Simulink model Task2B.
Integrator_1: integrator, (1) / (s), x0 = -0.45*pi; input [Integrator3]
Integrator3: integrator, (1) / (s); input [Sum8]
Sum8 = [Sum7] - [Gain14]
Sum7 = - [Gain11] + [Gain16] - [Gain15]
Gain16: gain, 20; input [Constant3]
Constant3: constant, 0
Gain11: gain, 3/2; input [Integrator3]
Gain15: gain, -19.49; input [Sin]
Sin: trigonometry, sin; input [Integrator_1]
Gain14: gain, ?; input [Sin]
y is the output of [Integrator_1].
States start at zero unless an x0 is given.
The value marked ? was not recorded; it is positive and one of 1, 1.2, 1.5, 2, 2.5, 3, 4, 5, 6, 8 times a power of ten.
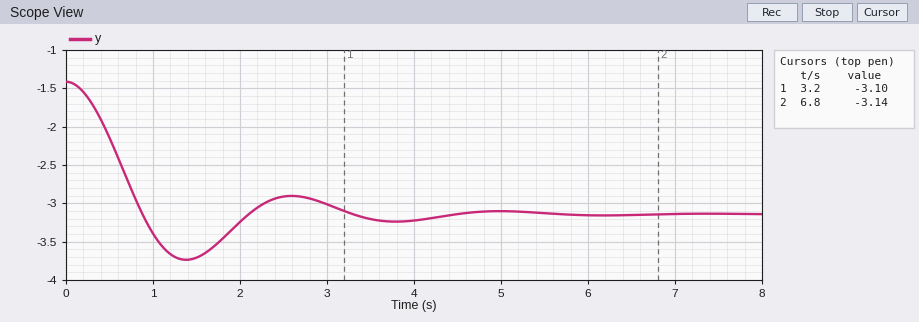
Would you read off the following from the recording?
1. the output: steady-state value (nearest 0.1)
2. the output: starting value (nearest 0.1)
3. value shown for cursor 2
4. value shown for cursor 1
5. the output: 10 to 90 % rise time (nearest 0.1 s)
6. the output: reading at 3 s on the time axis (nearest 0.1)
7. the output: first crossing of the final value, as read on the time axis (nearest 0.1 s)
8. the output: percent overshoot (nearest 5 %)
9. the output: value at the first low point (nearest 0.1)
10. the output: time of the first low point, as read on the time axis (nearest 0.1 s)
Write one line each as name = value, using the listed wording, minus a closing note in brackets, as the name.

the output: steady-state value = -3.1
the output: starting value = -1.4
value shown for cursor 2 = -3.14
value shown for cursor 1 = -3.10
the output: 10 to 90 % rise time = 0.6 s
the output: reading at 3 s on the time axis = -3.0
the output: first crossing of the final value, as read on the time axis = 0.9 s
the output: percent overshoot = 35 %
the output: value at the first low point = -3.7
the output: time of the first low point, as read on the time axis = 1.4 s
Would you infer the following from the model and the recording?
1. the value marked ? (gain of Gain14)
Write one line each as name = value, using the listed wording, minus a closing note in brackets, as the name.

the value marked ? = 12
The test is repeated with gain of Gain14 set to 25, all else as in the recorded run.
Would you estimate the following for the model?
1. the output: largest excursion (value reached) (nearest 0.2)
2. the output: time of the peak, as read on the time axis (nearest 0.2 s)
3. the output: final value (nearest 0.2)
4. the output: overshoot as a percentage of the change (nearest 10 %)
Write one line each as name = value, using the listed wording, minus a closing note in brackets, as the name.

the output: largest excursion (value reached) = 0.4
the output: time of the peak, as read on the time axis = 1.6 s
the output: final value = 0.0
the output: overshoot as a percentage of the change = 30 %
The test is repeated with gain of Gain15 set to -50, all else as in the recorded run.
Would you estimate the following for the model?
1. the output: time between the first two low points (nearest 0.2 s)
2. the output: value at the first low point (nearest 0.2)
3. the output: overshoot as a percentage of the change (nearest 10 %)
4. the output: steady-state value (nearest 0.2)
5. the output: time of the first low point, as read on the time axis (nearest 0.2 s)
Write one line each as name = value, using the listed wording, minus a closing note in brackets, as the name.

the output: time between the first two low points = 1.0 s
the output: value at the first low point = -4.2
the output: overshoot as a percentage of the change = 60 %
the output: steady-state value = -3.2
the output: time of the first low point, as read on the time axis = 0.6 s
